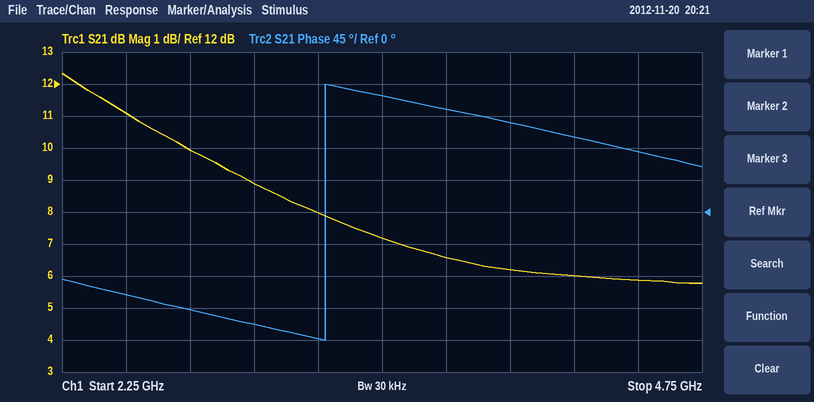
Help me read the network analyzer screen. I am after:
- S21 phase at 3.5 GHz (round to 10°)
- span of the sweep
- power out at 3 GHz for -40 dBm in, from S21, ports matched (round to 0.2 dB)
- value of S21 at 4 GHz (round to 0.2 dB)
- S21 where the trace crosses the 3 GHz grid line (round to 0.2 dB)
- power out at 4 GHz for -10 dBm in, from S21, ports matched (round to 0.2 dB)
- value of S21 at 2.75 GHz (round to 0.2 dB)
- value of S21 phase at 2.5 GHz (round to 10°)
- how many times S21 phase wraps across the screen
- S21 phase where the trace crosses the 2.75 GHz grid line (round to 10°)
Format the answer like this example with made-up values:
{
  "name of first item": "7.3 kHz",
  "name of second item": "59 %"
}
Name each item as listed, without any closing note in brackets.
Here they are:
{
  "S21 phase at 3.5 GHz": "160°",
  "span of the sweep": "2.5 GHz",
  "power out at 3 GHz for -40 dBm in, from S21, ports matched": "-31.2 dBm",
  "value of S21 at 4 GHz": "6.2 dB",
  "S21 where the trace crosses the 3 GHz grid line": "8.8 dB",
  "power out at 4 GHz for -10 dBm in, from S21, ports matched": "-3.8 dBm",
  "value of S21 at 2.75 GHz": "10.0 dB",
  "value of S21 phase at 2.5 GHz": "-120°",
  "how many times S21 phase wraps across the screen": "1",
  "S21 phase where the trace crosses the 2.75 GHz grid line": "-140°"
}
